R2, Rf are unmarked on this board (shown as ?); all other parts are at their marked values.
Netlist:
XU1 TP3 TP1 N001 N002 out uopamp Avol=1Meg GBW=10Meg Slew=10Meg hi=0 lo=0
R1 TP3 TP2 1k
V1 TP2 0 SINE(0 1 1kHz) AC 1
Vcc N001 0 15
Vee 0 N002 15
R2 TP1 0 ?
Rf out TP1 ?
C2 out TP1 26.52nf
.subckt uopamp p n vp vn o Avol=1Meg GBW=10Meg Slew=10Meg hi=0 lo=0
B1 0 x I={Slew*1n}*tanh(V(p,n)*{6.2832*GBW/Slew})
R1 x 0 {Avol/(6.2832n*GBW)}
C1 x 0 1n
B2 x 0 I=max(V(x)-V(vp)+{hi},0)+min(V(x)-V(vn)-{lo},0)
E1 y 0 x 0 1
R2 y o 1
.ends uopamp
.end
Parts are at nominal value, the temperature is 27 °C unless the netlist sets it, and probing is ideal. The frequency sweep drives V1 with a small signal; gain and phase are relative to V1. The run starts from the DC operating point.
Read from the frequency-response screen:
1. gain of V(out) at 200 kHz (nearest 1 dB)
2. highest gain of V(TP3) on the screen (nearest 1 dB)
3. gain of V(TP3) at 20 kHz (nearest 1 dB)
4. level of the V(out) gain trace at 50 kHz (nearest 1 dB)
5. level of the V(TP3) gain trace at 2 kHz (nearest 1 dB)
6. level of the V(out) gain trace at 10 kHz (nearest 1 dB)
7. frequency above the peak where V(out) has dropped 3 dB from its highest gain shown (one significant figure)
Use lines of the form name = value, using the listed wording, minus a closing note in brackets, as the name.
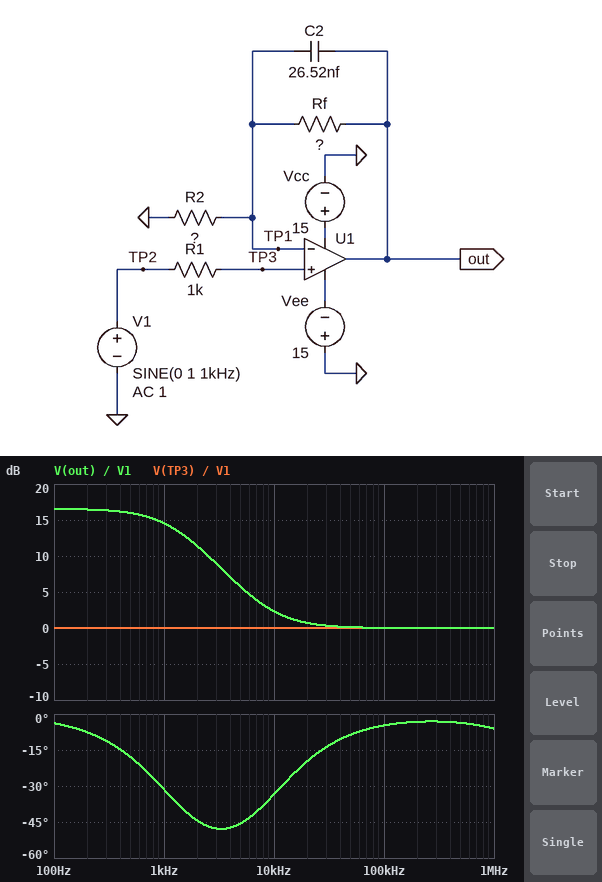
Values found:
gain of V(out) at 200 kHz = 0 dB
highest gain of V(TP3) on the screen = 0 dB
gain of V(TP3) at 20 kHz = 0 dB
level of the V(out) gain trace at 50 kHz = 0 dB
level of the V(TP3) gain trace at 2 kHz = 0 dB
level of the V(out) gain trace at 10 kHz = 2 dB
frequency above the peak where V(out) has dropped 3 dB from its highest gain shown = 1 kHz
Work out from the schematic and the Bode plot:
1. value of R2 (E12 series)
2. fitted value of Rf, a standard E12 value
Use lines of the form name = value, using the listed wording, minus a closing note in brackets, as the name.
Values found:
value of R2 = 820 Ω
fitted value of Rf, a standard E12 value = 4.7 kΩ
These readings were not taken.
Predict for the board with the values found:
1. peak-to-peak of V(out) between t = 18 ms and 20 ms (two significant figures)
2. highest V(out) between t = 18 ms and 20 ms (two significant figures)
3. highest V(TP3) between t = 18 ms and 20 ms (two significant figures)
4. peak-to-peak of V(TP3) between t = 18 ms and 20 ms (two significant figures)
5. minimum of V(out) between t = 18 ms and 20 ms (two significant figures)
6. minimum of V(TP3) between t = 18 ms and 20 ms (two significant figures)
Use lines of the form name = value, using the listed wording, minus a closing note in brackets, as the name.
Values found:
peak-to-peak of V(out) between t = 18 ms and 20 ms = 11 V
highest V(out) between t = 18 ms and 20 ms = 5.3 V
highest V(TP3) between t = 18 ms and 20 ms = 1.0 V
peak-to-peak of V(TP3) between t = 18 ms and 20 ms = 2.0 V
minimum of V(out) between t = 18 ms and 20 ms = -5.3 V
minimum of V(TP3) between t = 18 ms and 20 ms = -1.0 V
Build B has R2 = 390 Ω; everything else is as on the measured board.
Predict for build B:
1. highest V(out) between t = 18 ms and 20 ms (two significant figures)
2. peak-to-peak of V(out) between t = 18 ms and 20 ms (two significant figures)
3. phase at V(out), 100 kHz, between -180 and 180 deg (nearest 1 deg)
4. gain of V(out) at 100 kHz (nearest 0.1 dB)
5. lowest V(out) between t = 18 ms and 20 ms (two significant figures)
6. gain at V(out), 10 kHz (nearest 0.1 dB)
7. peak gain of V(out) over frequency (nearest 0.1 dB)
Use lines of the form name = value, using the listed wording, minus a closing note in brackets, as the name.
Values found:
highest V(out) between t = 18 ms and 20 ms = 10 V
peak-to-peak of V(out) between t = 18 ms and 20 ms = 21 V
phase at V(out), 100 kHz, between -180 and 180 deg = -9 deg
gain of V(out) at 100 kHz = 0.1 dB
lowest V(out) between t = 18 ms and 20 ms = -10 V
gain at V(out), 10 kHz = 5.7 dB
peak gain of V(out) over frequency = 22.3 dB
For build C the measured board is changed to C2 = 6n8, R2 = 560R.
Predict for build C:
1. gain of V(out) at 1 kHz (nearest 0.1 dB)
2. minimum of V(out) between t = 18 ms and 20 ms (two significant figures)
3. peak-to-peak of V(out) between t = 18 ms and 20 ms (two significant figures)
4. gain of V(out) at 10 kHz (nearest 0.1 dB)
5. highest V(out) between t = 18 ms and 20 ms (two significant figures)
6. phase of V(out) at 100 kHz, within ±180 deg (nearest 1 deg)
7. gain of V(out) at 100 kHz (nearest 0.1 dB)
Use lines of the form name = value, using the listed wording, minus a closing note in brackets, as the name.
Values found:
gain of V(out) at 1 kHz = 19.3 dB
minimum of V(out) between t = 18 ms and 20 ms = -9.2 V
peak-to-peak of V(out) between t = 18 ms and 20 ms = 18 V
gain of V(out) at 10 kHz = 12.6 dB
highest V(out) between t = 18 ms and 20 ms = 9.2 V
phase of V(out) at 100 kHz, within ±180 deg = -23 deg
gain of V(out) at 100 kHz = 0.8 dB
